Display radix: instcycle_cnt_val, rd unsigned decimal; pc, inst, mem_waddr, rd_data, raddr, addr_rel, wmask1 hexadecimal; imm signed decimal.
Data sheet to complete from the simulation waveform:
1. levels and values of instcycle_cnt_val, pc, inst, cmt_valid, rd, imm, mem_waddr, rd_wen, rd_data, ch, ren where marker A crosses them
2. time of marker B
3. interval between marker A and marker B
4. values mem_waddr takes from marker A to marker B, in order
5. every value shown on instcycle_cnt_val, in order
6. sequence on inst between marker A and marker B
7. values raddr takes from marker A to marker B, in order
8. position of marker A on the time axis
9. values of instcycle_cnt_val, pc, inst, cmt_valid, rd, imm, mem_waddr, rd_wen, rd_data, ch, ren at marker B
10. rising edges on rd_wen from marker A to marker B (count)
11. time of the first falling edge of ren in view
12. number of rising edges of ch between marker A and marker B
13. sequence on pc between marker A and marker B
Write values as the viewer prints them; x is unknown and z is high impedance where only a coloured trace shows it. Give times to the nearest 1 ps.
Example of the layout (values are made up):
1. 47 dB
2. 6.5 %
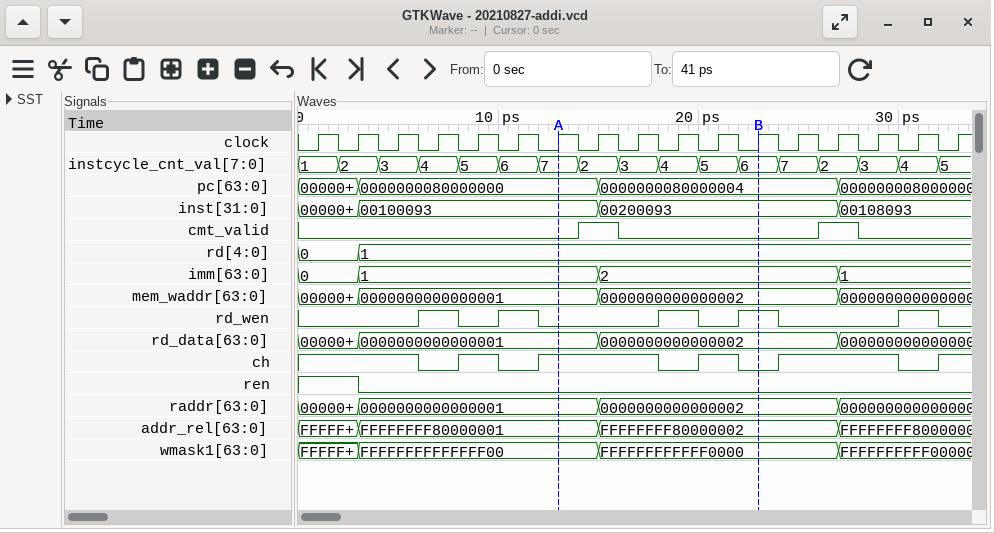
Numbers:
1. instcycle_cnt_val=7, pc=0000000080000000, inst=00100093, cmt_valid=0, rd=1, imm=1, mem_waddr=0000000000000001, rd_wen=0, rd_data=0000000000000001, ch=1, ren=0
2. 23 ps
3. 10 ps
4. 0000000000000001, 0000000000000002
5. 1, 2, 3, 4, 5, 6, 7, 2, 3, 4, 5, 6, 7, 2, 3, 4, 5
6. 00100093, 00200093
7. 0000000000000001, 0000000000000002
8. 13 ps
9. instcycle_cnt_val=6, pc=0000000080000004, inst=00200093, cmt_valid=0, rd=1, imm=2, mem_waddr=0000000000000002, rd_wen=1, rd_data=0000000000000002, ch=0, ren=0
10. 2
11. 3 ps
12. 1
13. 0000000080000000, 0000000080000004
